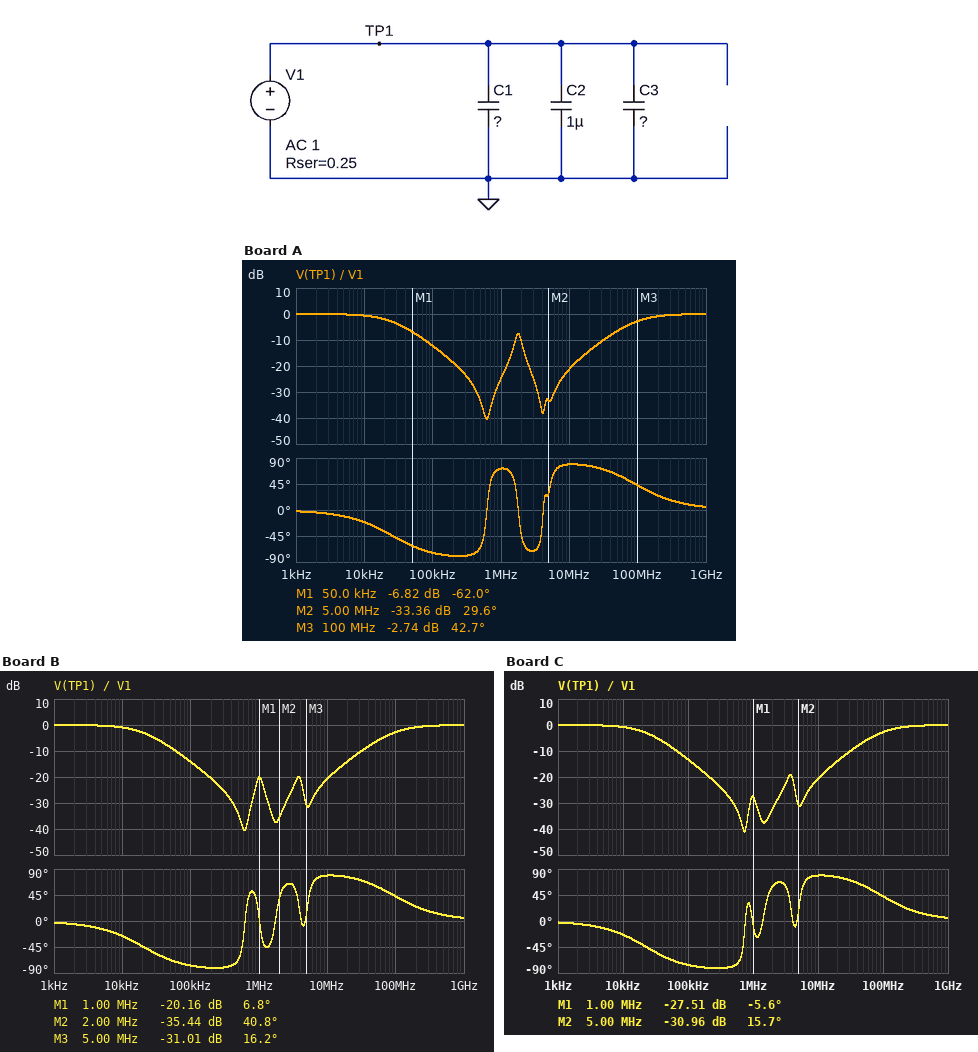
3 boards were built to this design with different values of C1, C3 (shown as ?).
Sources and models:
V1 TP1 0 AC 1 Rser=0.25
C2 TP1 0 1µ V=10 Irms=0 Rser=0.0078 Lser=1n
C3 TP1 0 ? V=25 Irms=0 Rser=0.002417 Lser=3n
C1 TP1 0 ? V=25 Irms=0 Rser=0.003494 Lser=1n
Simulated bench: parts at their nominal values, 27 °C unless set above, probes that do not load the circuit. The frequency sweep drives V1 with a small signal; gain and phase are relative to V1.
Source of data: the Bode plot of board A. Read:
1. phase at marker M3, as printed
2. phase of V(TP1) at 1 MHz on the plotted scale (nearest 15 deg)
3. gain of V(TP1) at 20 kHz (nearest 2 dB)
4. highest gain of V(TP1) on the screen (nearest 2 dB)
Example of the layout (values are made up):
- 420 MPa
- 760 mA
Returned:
- 42.7 deg
- 75 deg
- -2 dB
- 0 dB
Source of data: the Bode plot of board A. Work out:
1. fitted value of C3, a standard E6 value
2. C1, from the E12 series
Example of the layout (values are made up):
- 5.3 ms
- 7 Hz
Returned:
- 22 µF
- 1.5 µF
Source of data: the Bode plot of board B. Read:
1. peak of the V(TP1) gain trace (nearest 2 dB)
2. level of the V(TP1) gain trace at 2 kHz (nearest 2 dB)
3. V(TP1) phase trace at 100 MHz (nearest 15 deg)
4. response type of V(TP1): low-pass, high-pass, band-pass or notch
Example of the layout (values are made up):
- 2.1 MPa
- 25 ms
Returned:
- 0 dB
- 0 dB
- 45 deg
- notch
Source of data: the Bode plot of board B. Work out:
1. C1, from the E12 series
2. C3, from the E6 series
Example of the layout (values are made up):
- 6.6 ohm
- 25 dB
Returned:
- 8.2 µF
- 22 µF
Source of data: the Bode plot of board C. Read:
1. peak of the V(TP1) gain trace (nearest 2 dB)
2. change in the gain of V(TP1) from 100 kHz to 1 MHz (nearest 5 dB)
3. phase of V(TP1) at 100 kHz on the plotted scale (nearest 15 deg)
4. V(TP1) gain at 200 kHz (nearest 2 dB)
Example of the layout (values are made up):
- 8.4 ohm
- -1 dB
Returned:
- 0 dB
- -15 dB
- -75 deg
- -20 dB
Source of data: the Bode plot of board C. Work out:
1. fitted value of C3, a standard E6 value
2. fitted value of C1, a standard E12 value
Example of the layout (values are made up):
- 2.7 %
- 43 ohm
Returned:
- 15 µF
- 12 µF
